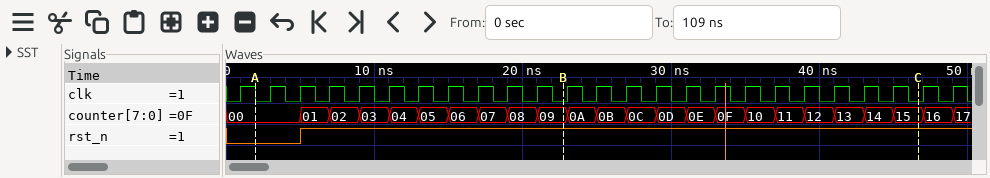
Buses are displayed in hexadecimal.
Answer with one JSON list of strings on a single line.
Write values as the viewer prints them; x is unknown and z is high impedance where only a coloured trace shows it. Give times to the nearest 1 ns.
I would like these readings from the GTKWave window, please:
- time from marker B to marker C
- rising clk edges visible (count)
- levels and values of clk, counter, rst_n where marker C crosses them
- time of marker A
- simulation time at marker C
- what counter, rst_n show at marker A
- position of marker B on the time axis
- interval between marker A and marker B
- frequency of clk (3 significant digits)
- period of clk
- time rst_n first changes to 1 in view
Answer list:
["24 ns", "25", "clk=0, counter=15, rst_n=1", "2 ns", "47 ns", "counter=00, rst_n=0", "23 ns", "21 ns", "500 MHz", "2 ns", "5 ns"]
